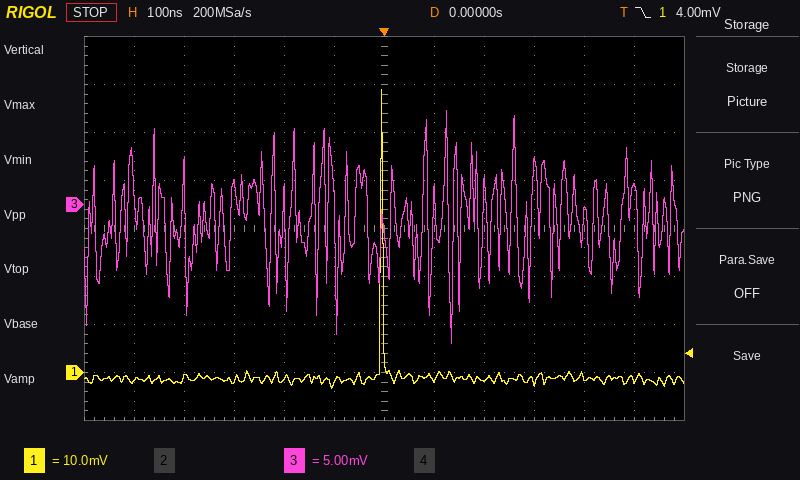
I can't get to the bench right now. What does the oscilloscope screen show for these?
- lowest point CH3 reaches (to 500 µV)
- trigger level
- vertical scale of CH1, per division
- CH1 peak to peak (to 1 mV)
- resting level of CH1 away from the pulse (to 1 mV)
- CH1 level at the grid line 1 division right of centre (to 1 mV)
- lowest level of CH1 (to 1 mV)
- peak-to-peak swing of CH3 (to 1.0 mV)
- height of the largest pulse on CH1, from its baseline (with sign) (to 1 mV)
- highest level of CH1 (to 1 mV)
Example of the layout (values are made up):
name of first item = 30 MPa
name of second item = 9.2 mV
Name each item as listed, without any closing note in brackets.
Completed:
lowest point CH3 reaches = -14.5 mV
trigger level = 4.00 mV
vertical scale of CH1, per division = 10 mV
CH1 peak to peak = 62 mV
resting level of CH1 away from the pulse = -1 mV
CH1 level at the grid line 1 division right of centre = -1 mV
lowest level of CH1 = -3 mV
peak-to-peak swing of CH3 = 24.0 mV
height of the largest pulse on CH1, from its baseline (with sign) = +60 mV
highest level of CH1 = 59 mV
